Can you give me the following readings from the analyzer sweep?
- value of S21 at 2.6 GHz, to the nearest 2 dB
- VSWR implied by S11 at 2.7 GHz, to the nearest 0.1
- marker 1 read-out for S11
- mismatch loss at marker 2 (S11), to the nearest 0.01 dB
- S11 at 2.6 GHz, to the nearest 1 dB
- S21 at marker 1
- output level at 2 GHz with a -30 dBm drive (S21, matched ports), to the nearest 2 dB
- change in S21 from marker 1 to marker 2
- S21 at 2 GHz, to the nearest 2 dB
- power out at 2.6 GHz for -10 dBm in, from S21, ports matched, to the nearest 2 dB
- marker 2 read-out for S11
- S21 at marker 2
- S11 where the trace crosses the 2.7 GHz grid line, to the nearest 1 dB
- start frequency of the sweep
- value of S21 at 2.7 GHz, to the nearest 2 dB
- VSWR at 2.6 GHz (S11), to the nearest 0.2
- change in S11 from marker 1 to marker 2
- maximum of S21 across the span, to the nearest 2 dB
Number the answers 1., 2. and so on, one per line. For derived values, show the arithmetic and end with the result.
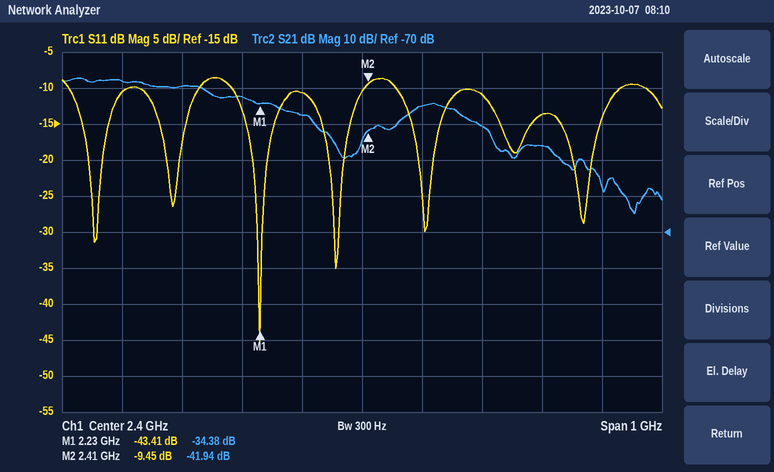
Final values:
1. -40 dB
2. |Γ| = 10^(-14/20) = 0.1995; VSWR = (1 + 0.1995)/(1 − 0.1995) ≈ 1.5
3. -43.41 dB
4. −10 log10(1 − 10^(-9.45/10)) ≈ 0.52 dB
5. -11 dB
6. -34.38 dB
7. -30 dBm + (-28 dB) = -58 dBm
8. -41.94 − (-34.38) = -7.56 dB
9. -28 dB
10. -10 dBm + (-40 dB) = -50 dBm
11. -9.45 dB
12. -41.94 dB
13. -14 dB
14. 1.9 GHz
15. -46 dB
16. |Γ| = 10^(-11/20) = 0.2818; VSWR = (1 + 0.2818)/(1 − 0.2818) ≈ 1.8
17. -9.45 − (-43.41) = 33.96 dB
18. -28 dB
